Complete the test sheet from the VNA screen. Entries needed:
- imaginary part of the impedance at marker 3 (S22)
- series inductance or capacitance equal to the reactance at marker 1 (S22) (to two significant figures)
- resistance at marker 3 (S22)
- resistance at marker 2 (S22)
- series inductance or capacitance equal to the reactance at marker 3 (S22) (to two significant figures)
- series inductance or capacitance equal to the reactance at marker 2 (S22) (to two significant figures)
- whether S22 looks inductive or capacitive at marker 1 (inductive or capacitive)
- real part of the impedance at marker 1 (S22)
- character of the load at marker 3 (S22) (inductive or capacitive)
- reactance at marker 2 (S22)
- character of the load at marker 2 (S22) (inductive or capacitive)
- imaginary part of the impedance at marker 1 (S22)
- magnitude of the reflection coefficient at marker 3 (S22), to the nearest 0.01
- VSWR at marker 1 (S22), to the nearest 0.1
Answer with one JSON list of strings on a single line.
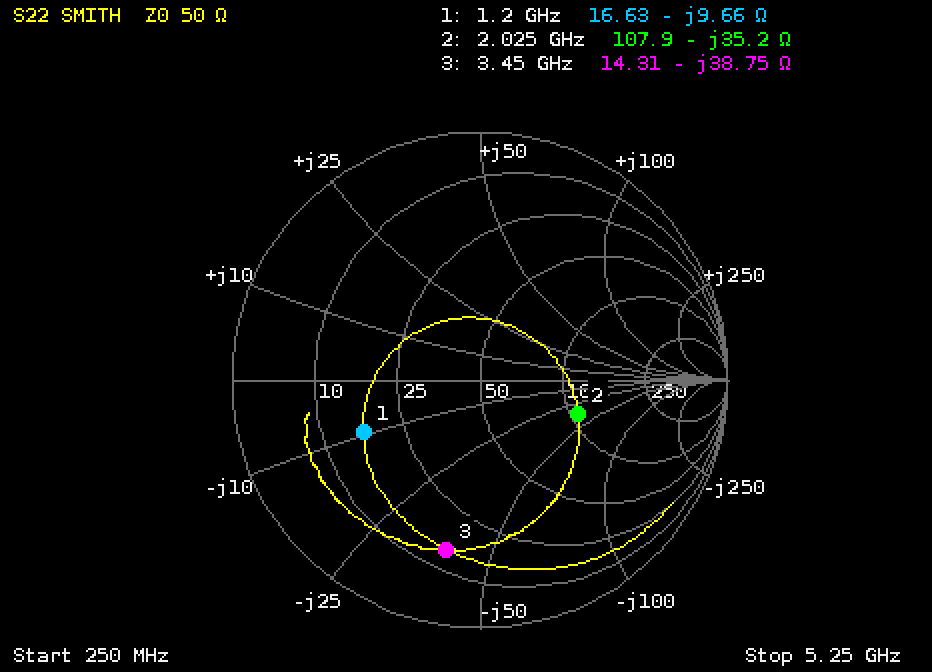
["-38.75 Ω", "14 pF", "14.31 Ω", "107.9 Ω", "1.2 pF", "2.2 pF", "capacitive", "16.63 Ω", "capacitive", "-35.2 Ω", "capacitive", "-9.66 Ω", "0.70", "3.1"]
